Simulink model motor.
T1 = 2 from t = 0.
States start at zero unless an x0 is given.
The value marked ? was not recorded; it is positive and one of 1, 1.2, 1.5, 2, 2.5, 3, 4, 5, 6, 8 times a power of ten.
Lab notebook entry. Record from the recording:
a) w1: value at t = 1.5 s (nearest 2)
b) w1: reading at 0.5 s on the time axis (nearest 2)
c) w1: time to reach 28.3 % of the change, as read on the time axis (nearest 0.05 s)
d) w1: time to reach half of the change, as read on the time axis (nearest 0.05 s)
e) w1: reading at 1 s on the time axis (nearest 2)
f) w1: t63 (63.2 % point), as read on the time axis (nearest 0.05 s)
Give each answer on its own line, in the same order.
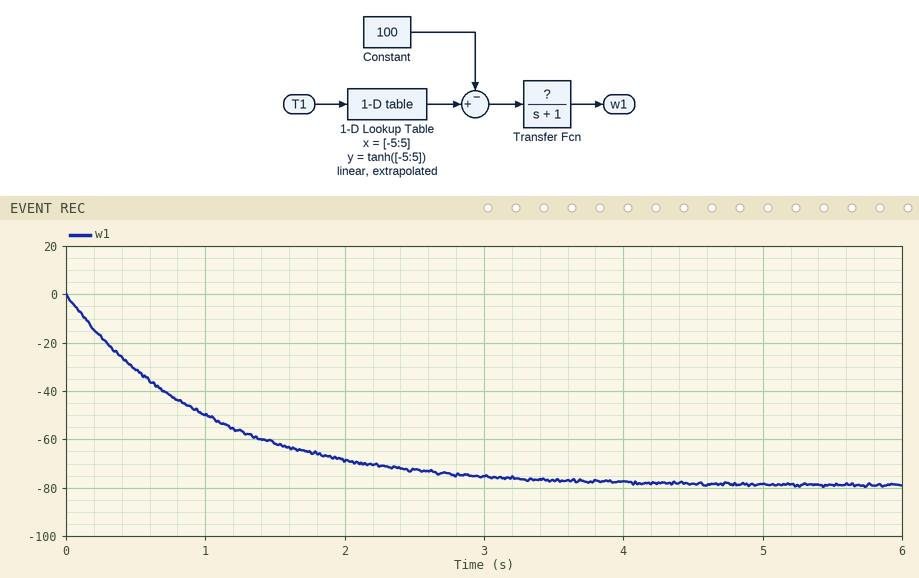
-62
-32
0.35 s
0.70 s
-50
1.00 s
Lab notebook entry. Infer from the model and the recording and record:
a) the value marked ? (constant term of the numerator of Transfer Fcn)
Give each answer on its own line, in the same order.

0.8
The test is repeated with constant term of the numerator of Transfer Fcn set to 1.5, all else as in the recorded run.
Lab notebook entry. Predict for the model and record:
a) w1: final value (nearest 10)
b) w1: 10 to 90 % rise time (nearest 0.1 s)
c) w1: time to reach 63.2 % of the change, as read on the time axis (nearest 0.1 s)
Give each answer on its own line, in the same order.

-150
2.2 s
1.0 s
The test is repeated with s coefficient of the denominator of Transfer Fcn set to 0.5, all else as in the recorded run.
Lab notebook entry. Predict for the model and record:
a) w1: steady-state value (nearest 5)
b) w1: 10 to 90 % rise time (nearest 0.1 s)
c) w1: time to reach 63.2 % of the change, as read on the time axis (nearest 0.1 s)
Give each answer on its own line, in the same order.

-80
1.1 s
0.5 s
